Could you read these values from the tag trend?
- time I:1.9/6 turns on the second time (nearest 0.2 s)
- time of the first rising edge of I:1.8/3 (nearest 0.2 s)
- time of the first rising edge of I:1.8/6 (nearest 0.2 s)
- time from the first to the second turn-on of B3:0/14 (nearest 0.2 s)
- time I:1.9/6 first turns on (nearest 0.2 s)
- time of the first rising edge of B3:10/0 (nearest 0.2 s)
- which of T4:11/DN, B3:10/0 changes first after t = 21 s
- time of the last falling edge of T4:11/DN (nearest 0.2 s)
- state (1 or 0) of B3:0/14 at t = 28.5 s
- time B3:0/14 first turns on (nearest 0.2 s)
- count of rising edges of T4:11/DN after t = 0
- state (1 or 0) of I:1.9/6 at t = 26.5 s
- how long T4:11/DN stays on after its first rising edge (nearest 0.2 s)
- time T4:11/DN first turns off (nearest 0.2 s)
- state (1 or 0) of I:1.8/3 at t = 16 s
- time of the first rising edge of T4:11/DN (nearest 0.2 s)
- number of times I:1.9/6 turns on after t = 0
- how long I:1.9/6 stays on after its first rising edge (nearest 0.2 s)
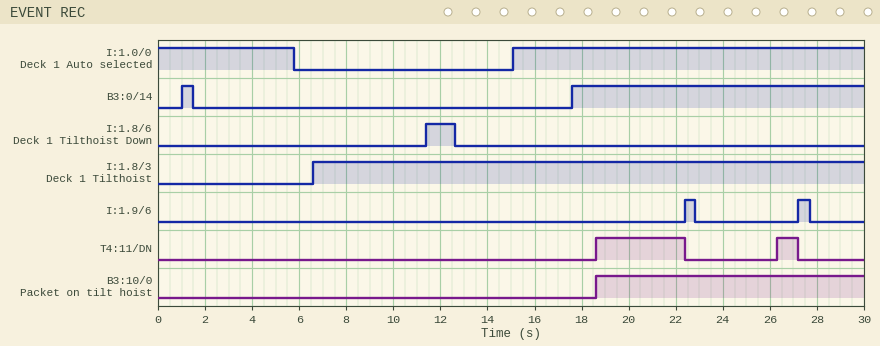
27.2 s
6.6 s
11.4 s
16.6 s
22.4 s
18.6 s
T4:11/DN
27.2 s
1
1.0 s
2
0
3.8 s
22.4 s
1
18.6 s
2
0.4 s
